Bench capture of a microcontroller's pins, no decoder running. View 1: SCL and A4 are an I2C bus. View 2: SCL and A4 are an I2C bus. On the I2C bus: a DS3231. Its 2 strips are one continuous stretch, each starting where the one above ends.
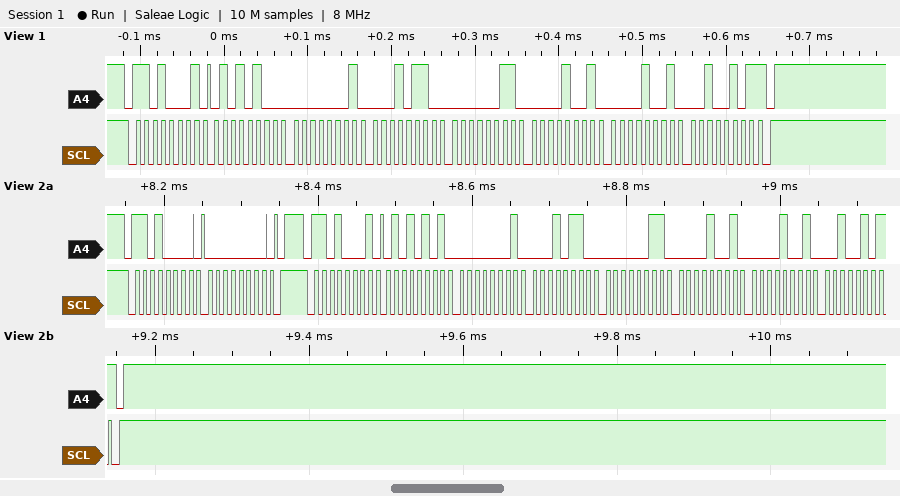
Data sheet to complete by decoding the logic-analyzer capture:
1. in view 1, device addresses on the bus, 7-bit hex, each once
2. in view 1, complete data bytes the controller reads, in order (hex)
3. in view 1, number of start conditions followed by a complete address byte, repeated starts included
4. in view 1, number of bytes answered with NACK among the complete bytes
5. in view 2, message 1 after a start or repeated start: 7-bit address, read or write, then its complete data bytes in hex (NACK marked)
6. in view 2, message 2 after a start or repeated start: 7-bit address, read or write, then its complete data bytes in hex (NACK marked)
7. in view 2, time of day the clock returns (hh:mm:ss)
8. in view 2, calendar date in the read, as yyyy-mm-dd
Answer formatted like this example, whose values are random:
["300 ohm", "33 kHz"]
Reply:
["0x68", "54 01 16 03 09 09 25", "1", "1", "0x68 write: 00", "0x68 read: 55 01 16 03 09 09 25 NACK", "16:01:55", "2025-09-09"]
